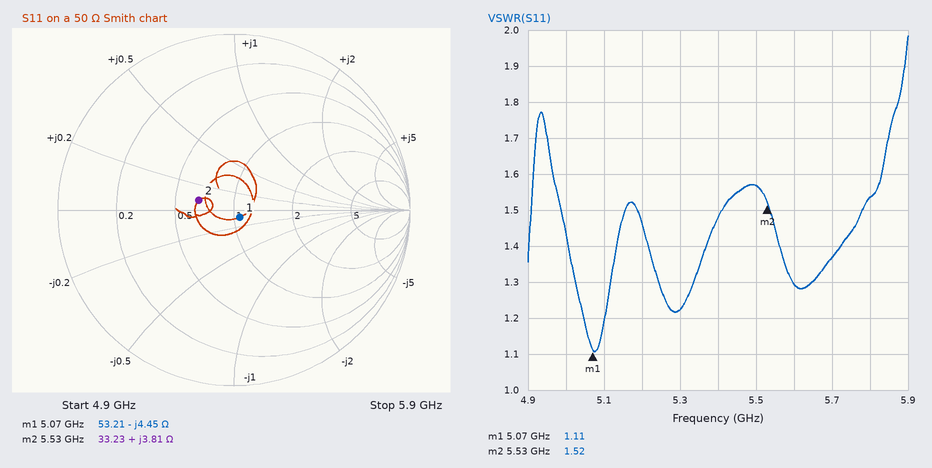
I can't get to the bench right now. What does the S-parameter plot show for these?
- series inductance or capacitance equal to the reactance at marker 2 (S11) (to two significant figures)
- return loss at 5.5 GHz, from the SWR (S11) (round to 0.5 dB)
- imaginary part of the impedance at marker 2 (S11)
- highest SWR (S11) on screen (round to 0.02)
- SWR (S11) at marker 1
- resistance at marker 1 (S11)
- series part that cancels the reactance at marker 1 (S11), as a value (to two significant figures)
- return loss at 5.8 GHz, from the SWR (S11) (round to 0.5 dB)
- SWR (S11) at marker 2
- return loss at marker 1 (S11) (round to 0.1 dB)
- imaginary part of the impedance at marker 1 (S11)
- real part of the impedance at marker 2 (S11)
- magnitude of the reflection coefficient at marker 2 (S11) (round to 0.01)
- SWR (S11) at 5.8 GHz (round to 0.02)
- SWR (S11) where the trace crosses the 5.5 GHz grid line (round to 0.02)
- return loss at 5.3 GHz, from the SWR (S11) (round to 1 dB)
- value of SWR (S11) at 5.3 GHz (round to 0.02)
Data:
110 pH
13.0 dB
+3.81 Ω
1.98
1.11
53.21 Ω
140 pH
13.5 dB
1.52
25.5 dB
-4.45 Ω
33.23 Ω
0.21
1.54
1.56
20 dB
1.22
